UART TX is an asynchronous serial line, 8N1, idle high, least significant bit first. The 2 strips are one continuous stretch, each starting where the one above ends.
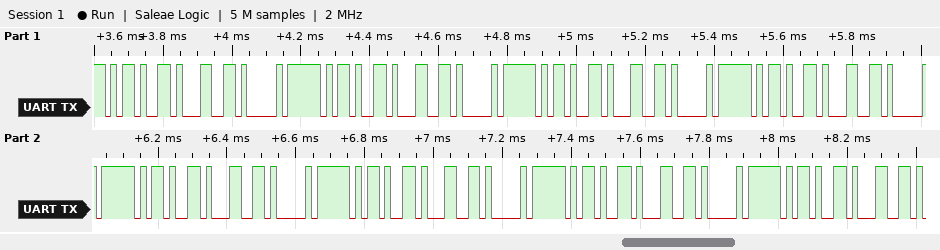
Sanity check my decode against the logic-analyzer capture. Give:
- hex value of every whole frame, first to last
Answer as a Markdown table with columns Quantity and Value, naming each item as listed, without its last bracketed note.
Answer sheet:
| Quantity | Value |
|---|---|
| hex value of every whole frame, first to last | 2D 31 41 2D 31 41 2D 31 41 2D 31 41 2D 31 41 2D 31 41 2D 31 41 2D 31 |
